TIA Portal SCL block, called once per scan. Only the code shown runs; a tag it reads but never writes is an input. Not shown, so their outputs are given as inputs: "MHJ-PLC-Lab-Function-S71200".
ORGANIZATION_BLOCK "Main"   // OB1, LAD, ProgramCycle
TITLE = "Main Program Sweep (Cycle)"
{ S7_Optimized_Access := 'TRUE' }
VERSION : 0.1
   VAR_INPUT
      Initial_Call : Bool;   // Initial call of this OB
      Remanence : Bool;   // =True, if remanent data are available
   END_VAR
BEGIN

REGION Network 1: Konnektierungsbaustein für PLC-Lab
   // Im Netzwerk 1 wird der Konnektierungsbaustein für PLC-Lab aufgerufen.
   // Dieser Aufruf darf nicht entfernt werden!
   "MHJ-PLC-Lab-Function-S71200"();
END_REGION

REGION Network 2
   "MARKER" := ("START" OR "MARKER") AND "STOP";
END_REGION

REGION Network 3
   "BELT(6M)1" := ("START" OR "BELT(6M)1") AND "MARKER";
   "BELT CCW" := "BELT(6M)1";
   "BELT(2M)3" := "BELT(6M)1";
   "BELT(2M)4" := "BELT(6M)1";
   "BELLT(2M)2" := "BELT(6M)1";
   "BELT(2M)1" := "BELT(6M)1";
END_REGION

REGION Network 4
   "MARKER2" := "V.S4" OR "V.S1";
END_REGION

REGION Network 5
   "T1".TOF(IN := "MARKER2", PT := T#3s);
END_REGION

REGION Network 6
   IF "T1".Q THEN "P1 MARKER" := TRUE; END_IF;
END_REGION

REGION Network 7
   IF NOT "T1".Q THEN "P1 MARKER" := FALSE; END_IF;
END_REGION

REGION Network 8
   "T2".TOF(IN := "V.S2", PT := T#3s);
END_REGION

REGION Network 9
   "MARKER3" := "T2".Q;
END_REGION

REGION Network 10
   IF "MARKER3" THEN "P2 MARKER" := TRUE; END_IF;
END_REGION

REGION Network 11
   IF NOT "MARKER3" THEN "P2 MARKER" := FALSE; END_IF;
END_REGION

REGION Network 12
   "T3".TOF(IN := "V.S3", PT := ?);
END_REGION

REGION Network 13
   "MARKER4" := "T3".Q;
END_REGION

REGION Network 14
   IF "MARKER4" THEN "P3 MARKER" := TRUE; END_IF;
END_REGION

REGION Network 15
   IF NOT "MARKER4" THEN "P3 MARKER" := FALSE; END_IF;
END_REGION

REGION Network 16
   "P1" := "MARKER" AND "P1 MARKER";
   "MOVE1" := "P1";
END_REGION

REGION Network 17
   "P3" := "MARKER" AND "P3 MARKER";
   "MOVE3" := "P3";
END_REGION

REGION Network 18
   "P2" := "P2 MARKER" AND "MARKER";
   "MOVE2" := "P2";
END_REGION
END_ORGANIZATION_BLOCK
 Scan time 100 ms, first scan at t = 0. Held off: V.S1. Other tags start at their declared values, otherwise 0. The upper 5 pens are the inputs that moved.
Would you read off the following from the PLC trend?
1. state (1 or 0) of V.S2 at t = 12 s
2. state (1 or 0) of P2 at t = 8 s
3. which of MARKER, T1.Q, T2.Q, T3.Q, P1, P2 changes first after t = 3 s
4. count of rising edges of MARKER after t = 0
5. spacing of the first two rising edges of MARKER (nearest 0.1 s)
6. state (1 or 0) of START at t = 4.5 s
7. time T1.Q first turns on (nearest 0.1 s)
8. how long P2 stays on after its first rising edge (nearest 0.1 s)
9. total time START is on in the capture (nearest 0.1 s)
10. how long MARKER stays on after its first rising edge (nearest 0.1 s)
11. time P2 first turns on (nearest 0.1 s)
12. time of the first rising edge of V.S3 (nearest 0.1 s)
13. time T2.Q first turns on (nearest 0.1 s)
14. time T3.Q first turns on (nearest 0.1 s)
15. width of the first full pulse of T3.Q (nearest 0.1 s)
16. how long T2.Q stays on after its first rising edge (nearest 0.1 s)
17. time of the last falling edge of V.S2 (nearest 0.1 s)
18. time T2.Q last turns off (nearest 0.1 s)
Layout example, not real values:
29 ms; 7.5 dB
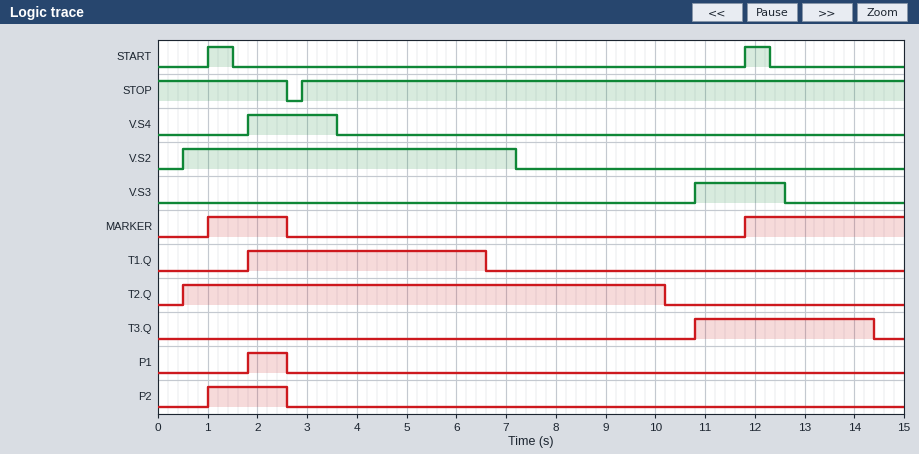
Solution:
0; 0; T1.Q; 2; 10.8 s; 0; 1.8 s; 1.6 s; 1.0 s; 1.6 s; 1.0 s; 10.8 s; 0.5 s; 10.8 s; 3.6 s; 9.7 s; 7.2 s; 10.2 s
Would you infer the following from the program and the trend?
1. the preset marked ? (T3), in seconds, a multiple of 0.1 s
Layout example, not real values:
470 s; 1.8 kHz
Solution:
1.8 s
